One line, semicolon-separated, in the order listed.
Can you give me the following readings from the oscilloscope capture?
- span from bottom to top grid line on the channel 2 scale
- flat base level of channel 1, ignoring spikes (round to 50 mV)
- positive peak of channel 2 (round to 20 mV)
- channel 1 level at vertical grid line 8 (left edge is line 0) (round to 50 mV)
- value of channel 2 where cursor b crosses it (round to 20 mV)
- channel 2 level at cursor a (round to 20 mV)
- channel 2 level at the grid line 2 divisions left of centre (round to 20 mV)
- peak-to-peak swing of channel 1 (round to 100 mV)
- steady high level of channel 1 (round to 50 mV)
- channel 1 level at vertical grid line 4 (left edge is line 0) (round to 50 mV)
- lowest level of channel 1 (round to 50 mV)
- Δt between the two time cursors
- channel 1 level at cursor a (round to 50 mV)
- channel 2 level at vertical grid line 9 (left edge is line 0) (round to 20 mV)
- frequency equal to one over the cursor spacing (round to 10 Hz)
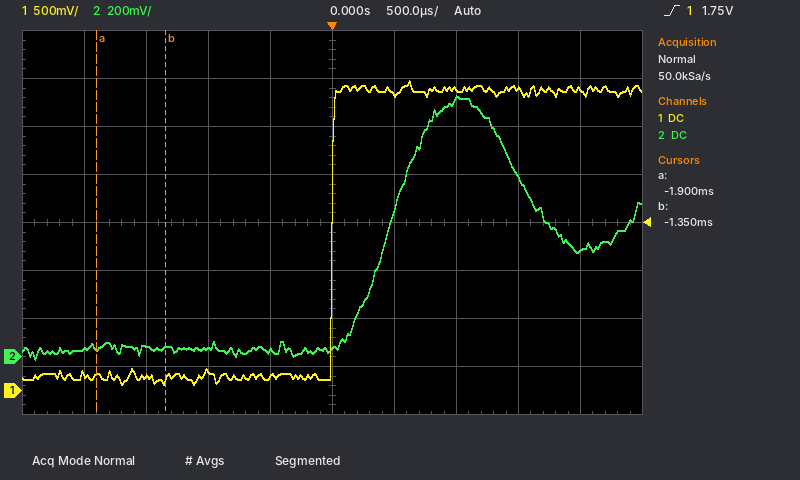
1.6 V; 150 mV; 1.08 V; 3.15 V; 40 mV; 40 mV; 40 mV; 3.20 V; 3.15 V; 150 mV; 50 mV; 550 µs; 150 mV; 440 mV; 1.82 kHz
